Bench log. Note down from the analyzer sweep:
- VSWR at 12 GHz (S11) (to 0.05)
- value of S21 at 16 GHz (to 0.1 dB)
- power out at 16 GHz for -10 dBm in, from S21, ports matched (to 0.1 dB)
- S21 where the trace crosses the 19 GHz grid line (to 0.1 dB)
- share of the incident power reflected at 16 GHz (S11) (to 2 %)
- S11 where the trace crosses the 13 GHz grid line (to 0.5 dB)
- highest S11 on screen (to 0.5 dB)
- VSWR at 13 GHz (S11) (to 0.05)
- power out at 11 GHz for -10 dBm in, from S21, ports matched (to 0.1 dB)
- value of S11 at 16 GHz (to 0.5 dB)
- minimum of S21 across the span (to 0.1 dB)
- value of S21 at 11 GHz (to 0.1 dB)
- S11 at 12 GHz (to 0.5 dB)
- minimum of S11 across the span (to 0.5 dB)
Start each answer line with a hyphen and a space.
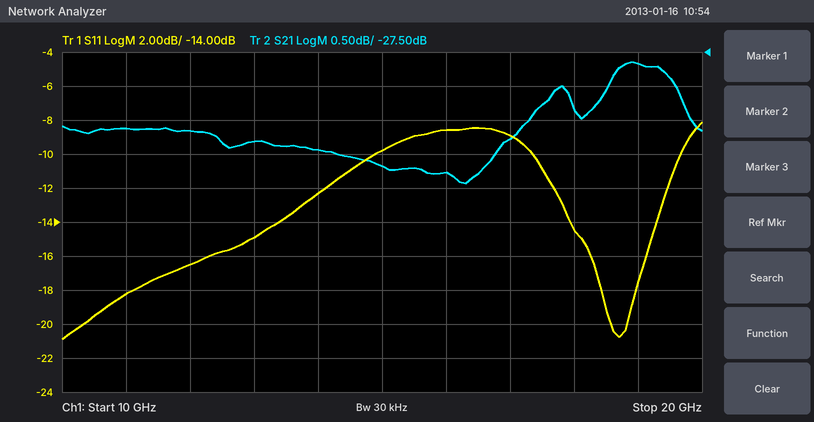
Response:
- 1.35
- -29.3 dB
- -39.3 dBm
- -27.7 dB
- 14 %
- -15.0 dB
- -8.0 dB
- 1.45
- -38.6 dBm
- -8.5 dB
- -29.4 dB
- -28.6 dB
- -16.5 dB
- -21.0 dB
